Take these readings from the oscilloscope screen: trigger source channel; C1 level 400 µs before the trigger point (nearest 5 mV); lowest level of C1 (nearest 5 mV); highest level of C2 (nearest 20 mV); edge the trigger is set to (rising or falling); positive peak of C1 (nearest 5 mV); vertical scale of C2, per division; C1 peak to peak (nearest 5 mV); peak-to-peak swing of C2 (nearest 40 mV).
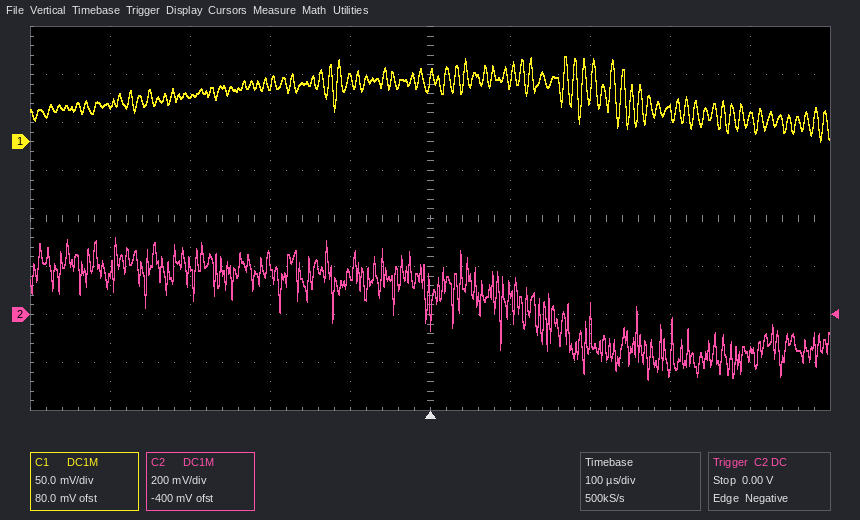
C2
40 mV
0 mV
320 mV
falling
90 mV
200 mV
90 mV
600 mV
